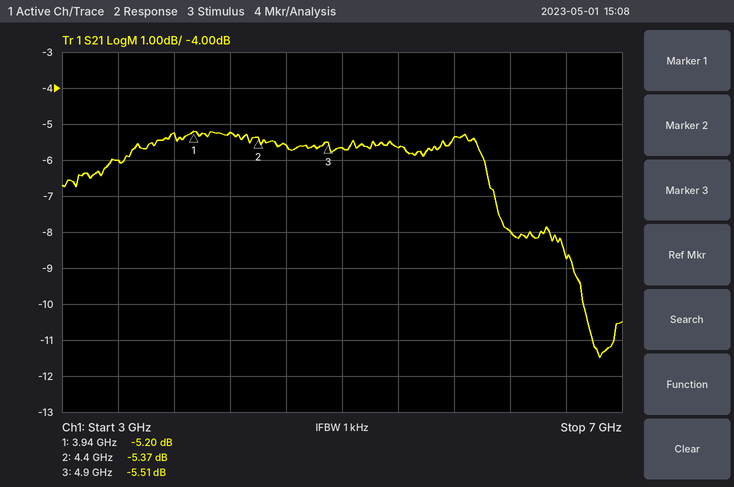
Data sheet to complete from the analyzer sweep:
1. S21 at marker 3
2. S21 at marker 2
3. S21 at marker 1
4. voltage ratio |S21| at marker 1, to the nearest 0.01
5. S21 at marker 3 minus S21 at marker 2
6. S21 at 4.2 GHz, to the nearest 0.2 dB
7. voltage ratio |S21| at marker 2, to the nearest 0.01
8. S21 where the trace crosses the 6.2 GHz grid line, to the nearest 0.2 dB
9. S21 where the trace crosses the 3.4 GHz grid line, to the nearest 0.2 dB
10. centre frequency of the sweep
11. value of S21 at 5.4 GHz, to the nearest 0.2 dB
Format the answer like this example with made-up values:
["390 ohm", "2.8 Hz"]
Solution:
["-5.51 dB", "-5.37 dB", "-5.20 dB", "0.55", "-0.14 dB", "-5.2 dB", "0.54", "-8.0 dB", "-6.0 dB", "5 GHz", "-5.6 dB"]
